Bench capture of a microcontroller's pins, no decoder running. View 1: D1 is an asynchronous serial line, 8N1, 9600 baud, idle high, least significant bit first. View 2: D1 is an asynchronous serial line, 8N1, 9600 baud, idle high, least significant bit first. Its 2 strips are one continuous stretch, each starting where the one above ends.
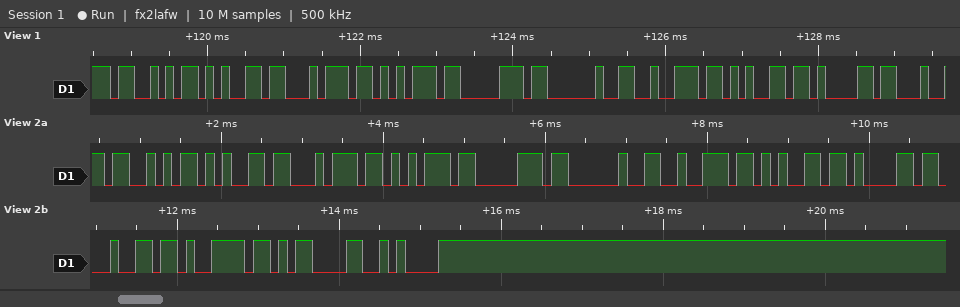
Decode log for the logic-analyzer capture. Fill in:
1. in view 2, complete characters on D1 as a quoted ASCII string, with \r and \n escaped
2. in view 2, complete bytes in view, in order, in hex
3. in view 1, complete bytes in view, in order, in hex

"Setup ready\r\n"
0x53 0x65 0x74 0x75 0x70 0x20 0x72 0x65 0x61 0x64 0x79 0x0D 0x0A
0x53 0x65 0x74 0x75 0x70 0x20 0x72 0x65 0x61
